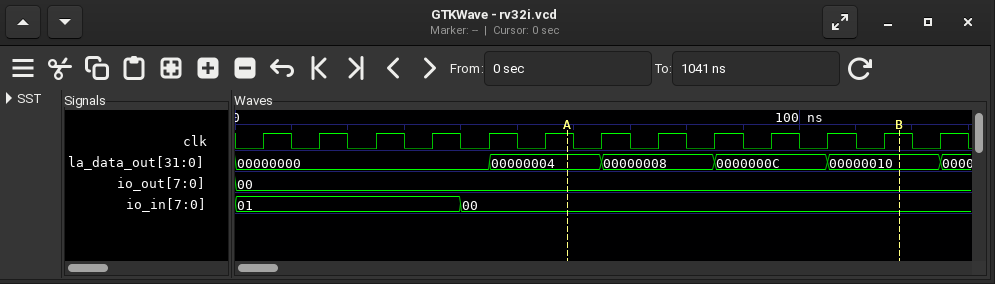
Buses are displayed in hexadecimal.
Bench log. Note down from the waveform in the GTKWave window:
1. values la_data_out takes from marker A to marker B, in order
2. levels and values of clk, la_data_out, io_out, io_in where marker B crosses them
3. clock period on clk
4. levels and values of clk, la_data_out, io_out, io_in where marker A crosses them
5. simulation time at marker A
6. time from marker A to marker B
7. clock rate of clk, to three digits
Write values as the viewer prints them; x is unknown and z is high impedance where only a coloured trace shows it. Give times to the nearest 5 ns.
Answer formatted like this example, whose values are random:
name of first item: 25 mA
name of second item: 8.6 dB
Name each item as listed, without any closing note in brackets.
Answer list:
values la_data_out takes from marker A to marker B, in order: 00000004, 00000008, 0000000C, 00000010
levels and values of clk, la_data_out, io_out, io_in where marker B crosses them: clk=1, la_data_out=00000010, io_out=00, io_in=00
clock period on clk: 10 ns
levels and values of clk, la_data_out, io_out, io_in where marker A crosses them: clk=1, la_data_out=00000004, io_out=00, io_in=00
simulation time at marker A: 60 ns
time from marker A to marker B: 60 ns
clock rate of clk, to three digits: 100 MHz
